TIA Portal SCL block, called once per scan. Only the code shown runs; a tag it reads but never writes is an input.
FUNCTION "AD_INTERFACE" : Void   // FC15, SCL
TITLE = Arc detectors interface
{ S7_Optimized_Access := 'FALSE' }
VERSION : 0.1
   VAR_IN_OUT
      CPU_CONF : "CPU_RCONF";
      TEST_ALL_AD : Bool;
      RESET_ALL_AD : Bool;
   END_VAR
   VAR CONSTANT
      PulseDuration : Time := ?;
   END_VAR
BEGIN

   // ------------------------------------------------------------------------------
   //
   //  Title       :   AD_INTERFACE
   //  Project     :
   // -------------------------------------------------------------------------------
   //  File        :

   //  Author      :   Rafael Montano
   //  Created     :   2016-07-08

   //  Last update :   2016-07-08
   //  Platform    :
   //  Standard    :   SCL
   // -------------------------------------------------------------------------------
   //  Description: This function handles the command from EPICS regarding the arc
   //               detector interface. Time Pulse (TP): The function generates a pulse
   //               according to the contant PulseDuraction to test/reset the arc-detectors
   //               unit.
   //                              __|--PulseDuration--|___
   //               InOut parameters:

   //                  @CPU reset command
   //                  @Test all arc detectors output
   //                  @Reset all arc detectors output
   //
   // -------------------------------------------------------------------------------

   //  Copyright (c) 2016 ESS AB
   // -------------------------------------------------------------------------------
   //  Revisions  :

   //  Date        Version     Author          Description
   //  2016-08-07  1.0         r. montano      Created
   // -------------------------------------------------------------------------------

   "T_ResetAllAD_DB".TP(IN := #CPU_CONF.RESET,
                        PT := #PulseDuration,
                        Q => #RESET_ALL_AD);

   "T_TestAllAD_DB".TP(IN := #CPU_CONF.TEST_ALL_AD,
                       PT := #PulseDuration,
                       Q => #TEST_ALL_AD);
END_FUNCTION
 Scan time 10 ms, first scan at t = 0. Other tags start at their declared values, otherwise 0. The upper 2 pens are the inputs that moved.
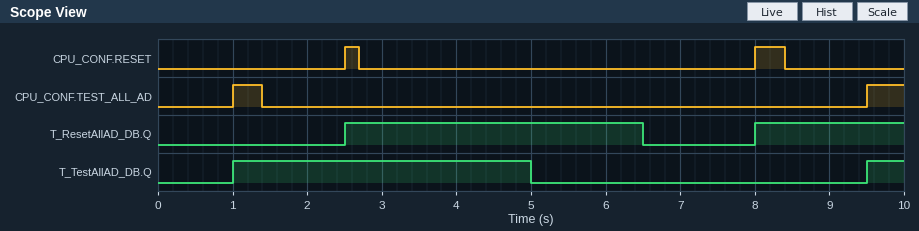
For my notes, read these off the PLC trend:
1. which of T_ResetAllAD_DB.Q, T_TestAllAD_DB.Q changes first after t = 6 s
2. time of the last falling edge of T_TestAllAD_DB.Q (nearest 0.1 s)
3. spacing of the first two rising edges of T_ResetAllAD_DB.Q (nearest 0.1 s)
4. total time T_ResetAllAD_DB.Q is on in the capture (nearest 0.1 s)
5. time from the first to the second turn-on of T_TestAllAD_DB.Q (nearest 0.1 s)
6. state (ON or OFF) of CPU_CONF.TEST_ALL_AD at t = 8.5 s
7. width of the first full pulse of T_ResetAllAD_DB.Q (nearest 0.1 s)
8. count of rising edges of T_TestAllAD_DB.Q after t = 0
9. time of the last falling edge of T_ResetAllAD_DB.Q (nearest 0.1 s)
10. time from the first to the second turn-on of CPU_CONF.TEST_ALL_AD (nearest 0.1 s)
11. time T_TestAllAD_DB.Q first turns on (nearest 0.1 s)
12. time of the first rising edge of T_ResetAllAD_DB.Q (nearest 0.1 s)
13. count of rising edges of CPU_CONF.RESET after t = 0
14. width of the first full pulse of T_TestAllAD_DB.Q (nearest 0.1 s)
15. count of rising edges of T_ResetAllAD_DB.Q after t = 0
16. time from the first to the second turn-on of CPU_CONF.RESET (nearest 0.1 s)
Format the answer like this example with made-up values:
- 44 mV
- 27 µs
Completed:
- T_ResetAllAD_DB.Q
- 5.0 s
- 5.5 s
- 6.0 s
- 8.5 s
- OFF
- 4.0 s
- 2
- 6.5 s
- 8.5 s
- 1.0 s
- 2.5 s
- 2
- 4.0 s
- 2
- 5.5 s
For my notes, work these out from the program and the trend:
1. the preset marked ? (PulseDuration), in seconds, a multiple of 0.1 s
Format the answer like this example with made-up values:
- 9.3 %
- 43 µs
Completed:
- 4.0 s
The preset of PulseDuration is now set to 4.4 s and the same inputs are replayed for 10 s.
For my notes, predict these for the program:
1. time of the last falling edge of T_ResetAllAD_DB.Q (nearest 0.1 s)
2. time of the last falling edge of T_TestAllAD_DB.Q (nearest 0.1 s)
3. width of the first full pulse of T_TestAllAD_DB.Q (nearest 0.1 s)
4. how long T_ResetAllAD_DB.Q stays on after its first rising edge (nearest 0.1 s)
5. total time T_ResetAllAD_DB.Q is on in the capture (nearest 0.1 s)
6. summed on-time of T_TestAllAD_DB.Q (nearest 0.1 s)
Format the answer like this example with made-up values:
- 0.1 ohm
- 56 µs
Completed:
- 6.9 s
- 5.4 s
- 4.4 s
- 4.4 s
- 6.4 s
- 4.9 s
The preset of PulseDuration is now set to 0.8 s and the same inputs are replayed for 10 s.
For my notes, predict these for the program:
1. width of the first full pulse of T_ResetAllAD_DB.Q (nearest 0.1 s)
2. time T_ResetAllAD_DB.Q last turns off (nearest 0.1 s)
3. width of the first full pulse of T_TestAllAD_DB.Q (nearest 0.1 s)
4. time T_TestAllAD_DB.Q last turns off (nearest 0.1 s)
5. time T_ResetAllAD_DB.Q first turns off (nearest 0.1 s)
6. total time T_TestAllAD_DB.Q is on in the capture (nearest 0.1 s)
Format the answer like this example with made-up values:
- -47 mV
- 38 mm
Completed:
- 0.8 s
- 8.8 s
- 0.8 s
- 1.8 s
- 3.3 s
- 1.3 s
